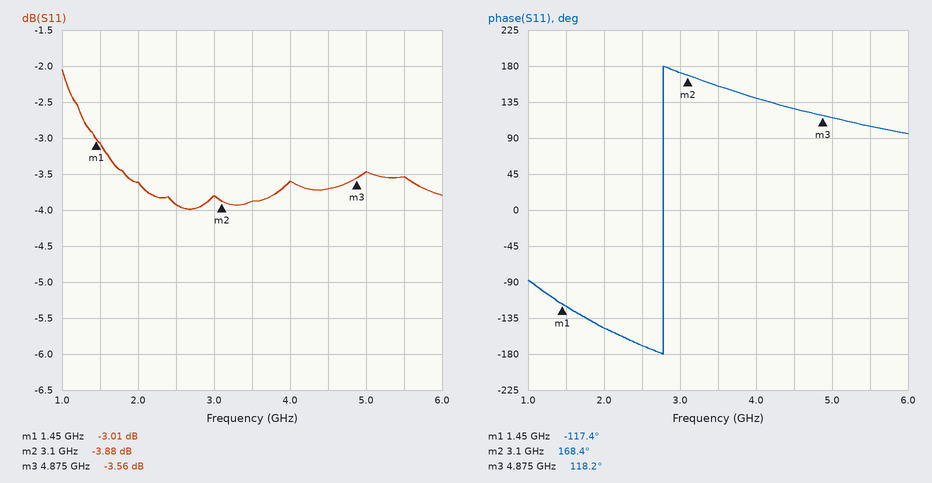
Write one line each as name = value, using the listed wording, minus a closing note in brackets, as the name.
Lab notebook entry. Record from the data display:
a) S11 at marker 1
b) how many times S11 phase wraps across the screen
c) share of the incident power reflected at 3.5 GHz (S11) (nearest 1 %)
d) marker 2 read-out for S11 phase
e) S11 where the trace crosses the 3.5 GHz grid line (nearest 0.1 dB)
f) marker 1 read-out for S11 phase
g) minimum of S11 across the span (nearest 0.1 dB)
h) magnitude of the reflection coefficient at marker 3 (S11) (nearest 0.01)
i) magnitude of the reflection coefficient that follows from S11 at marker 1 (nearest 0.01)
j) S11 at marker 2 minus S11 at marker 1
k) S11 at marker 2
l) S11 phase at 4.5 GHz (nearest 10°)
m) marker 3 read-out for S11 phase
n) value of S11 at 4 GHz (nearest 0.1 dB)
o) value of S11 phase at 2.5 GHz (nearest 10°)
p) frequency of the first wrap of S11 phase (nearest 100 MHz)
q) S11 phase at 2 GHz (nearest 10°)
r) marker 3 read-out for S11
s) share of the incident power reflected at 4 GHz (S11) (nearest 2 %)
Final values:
S11 at marker 1 = -3.01 dB
how many times S11 phase wraps across the screen = 1
share of the incident power reflected at 3.5 GHz (S11) = 41 %
marker 2 read-out for S11 phase = 168.4°
S11 where the trace crosses the 3.5 GHz grid line = -3.9 dB
marker 1 read-out for S11 phase = -117.4°
minimum of S11 across the span = -4.0 dB
magnitude of the reflection coefficient at marker 3 (S11) = 0.66
magnitude of the reflection coefficient that follows from S11 at marker 1 = 0.71
S11 at marker 2 minus S11 at marker 1 = -0.87 dB
S11 at marker 2 = -3.88 dB
S11 phase at 4.5 GHz = 130°
marker 3 read-out for S11 phase = 118.2°
value of S11 at 4 GHz = -3.6 dB
value of S11 phase at 2.5 GHz = -170°
frequency of the first wrap of S11 phase = 2.8 GHz
S11 phase at 2 GHz = -150°
marker 3 read-out for S11 = -3.56 dB
share of the incident power reflected at 4 GHz (S11) = 44 %
